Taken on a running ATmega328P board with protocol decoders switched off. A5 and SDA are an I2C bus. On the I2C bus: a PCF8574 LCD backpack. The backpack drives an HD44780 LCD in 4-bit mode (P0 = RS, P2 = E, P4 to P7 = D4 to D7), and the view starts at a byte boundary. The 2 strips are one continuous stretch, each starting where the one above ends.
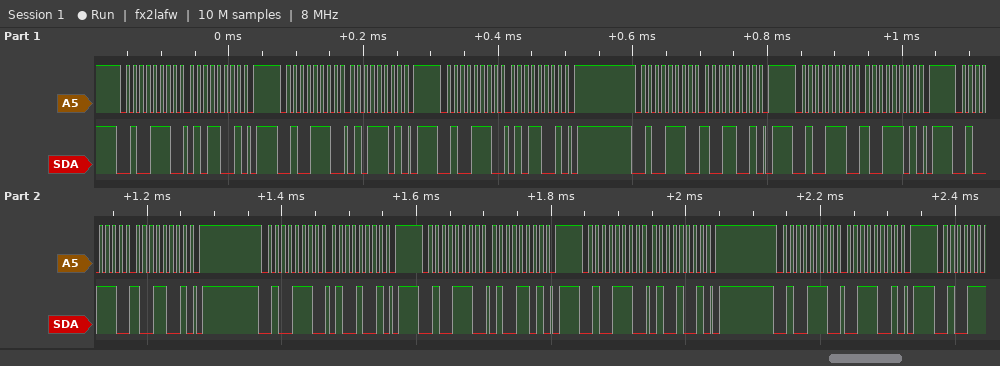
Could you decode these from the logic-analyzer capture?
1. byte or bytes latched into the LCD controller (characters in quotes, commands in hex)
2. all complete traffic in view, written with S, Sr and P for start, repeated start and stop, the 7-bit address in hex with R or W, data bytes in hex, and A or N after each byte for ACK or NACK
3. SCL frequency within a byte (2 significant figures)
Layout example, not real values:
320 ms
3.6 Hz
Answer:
'Y'
S 27W A 59 A P S 27W A 5D A P S 27W A 59 A P S 27W A 99 A P S 27W A 9D A P S 27W A 99 A P S 27W A 49 A P S 27W A 4D A P S 27W A 49 A P S 27W A 39 A P
100 kHz
